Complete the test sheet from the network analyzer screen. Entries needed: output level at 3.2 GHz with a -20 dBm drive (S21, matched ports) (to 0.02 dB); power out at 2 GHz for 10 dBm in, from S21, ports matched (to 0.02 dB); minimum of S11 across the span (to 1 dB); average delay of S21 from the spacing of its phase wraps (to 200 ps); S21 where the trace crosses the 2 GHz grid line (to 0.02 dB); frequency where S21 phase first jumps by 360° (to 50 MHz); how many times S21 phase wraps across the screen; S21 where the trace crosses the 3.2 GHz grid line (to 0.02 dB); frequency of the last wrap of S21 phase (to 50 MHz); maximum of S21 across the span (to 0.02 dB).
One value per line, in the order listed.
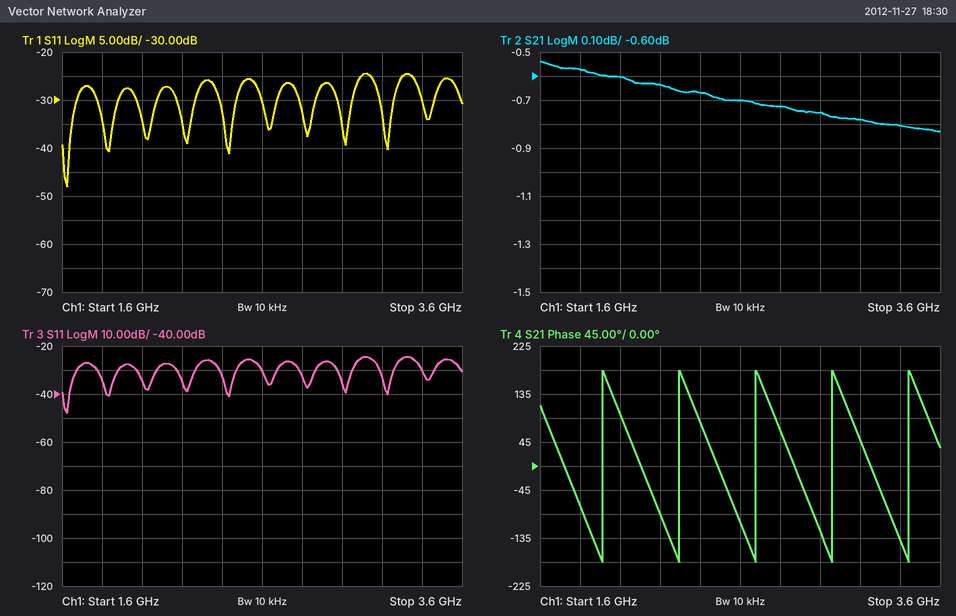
-20.78 dBm
9.40 dBm
-48 dB
2.6 ns
-0.60 dB
1.90 GHz
5
-0.78 dB
3.45 GHz
-0.54 dB
